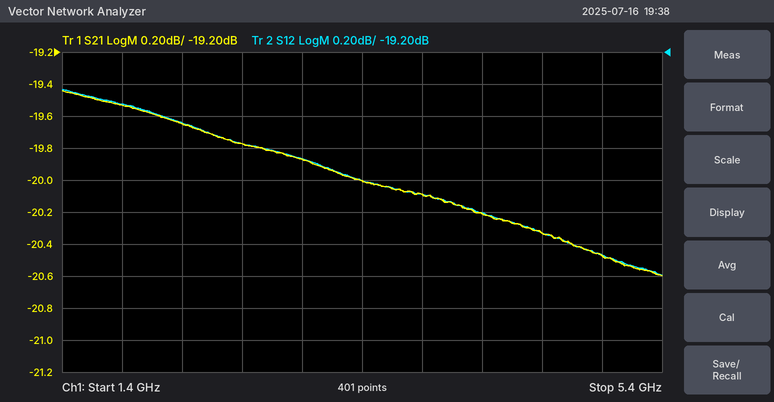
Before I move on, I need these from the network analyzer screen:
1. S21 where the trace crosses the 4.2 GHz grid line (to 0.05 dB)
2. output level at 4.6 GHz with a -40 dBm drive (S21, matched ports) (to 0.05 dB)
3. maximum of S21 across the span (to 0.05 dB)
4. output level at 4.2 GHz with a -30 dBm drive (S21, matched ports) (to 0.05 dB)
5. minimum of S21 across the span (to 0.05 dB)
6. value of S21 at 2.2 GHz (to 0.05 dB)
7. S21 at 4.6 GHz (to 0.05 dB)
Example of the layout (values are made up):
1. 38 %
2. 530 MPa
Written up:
1. -20.20 dB
2. -60.35 dBm
3. -19.45 dB
4. -50.20 dBm
5. -20.60 dB
6. -19.65 dB
7. -20.35 dB
